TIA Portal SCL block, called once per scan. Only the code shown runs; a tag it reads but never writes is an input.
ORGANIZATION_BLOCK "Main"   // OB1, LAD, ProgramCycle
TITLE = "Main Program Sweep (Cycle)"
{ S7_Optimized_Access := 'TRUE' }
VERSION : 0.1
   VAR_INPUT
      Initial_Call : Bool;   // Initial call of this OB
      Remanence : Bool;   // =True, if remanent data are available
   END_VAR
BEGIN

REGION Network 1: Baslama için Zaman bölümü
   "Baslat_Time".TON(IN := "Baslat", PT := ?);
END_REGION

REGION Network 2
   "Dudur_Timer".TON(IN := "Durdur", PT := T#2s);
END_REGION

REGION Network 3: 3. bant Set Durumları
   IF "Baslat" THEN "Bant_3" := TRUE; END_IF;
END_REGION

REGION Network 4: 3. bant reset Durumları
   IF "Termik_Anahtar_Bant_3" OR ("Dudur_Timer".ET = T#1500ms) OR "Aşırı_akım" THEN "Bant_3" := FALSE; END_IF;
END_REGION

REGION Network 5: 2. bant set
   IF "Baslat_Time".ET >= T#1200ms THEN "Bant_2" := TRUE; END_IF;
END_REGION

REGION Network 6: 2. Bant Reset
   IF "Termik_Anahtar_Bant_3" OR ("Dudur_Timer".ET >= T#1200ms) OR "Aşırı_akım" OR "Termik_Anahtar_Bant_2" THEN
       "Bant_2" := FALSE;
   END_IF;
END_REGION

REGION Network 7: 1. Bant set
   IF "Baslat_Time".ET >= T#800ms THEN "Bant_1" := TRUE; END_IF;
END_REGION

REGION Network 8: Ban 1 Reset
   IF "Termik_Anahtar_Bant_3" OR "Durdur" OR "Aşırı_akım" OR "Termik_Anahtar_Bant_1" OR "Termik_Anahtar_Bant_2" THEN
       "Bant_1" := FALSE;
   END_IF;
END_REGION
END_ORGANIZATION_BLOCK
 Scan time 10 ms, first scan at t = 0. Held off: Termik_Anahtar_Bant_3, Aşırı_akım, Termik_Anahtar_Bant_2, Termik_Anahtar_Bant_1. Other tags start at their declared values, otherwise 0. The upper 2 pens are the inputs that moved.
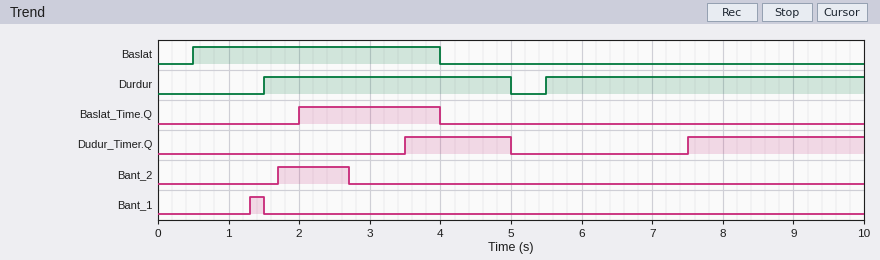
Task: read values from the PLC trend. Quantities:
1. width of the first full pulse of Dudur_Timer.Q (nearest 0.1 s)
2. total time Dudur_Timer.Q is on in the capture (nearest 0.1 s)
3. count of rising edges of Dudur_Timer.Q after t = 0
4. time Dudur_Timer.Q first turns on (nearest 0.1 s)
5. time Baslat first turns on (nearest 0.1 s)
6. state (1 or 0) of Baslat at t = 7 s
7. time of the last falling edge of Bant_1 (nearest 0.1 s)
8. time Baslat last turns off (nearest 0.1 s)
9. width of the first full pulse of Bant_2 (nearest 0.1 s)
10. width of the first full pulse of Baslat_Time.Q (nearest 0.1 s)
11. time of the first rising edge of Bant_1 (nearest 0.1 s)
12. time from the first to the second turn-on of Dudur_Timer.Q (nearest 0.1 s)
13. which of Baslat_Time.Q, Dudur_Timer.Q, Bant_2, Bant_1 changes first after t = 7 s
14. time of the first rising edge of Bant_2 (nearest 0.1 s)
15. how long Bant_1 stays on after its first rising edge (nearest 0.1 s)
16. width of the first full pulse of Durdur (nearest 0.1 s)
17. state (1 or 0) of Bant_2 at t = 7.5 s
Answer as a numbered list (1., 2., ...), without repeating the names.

1. 1.5 s
2. 4.0 s
3. 2
4. 3.5 s
5. 0.5 s
6. 0
7. 1.5 s
8. 4.0 s
9. 1.0 s
10. 2.0 s
11. 1.3 s
12. 4.0 s
13. Dudur_Timer.Q
14. 1.7 s
15. 0.2 s
16. 3.5 s
17. 0
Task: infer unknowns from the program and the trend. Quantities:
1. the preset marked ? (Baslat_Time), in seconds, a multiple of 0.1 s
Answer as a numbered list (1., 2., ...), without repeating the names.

1. 1.5 s
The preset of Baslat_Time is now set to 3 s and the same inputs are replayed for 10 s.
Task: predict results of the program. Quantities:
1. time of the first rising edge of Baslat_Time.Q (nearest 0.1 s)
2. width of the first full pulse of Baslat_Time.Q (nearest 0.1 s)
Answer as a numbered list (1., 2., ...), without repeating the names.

1. 3.5 s
2. 0.5 s
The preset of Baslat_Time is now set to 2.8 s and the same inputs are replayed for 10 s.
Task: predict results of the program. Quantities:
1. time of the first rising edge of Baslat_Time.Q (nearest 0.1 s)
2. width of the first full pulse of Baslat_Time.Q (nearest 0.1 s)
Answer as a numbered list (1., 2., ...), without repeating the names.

1. 3.3 s
2. 0.7 s
